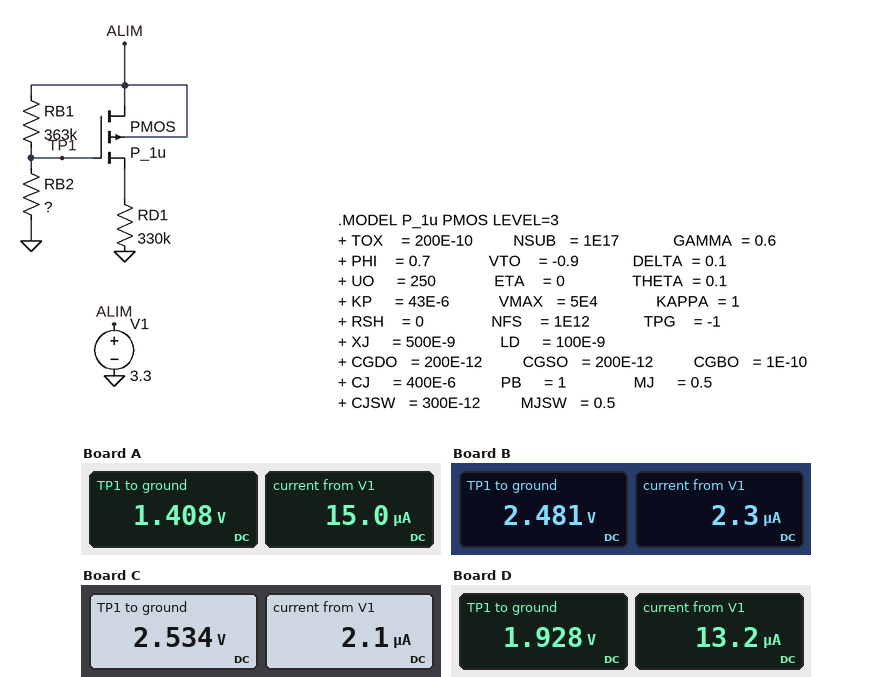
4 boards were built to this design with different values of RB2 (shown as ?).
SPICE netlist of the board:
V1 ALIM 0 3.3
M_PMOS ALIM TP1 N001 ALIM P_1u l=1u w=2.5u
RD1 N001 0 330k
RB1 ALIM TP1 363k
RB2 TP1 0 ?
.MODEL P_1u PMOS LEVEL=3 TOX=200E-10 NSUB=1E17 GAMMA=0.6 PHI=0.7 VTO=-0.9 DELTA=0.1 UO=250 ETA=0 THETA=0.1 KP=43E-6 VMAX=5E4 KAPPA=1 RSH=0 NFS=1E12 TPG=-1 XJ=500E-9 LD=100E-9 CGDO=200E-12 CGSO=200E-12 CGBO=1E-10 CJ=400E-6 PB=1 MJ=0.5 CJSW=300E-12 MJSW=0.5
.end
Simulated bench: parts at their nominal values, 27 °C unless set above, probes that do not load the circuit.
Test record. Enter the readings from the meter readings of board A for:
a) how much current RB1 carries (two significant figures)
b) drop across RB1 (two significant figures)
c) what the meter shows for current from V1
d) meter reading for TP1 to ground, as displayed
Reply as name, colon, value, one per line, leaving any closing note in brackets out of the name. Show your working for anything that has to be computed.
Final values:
how much current RB1 carries: (3.3 V - 1.408 V) / 363 kΩ = 5.2 µA
drop across RB1: 3.3 V - 1.408 V = 1.9 V
what the meter shows for current from V1: 15.0 µA
meter reading for TP1 to ground, as displayed: 1.408 V
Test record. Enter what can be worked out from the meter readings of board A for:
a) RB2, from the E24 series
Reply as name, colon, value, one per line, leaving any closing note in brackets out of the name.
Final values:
RB2, from the E24 series: 270 kΩ
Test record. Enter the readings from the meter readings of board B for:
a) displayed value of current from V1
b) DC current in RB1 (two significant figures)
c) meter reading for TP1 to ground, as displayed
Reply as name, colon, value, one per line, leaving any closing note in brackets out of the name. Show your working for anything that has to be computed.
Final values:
displayed value of current from V1: 2.3 µA
DC current in RB1: (3.3 V - 2.481 V) / 363 kΩ = 2.3 µA
meter reading for TP1 to ground, as displayed: 2.481 V
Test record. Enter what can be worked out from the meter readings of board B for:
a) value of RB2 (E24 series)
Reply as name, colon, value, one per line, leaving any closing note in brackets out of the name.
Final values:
value of RB2: 1.1 MΩ
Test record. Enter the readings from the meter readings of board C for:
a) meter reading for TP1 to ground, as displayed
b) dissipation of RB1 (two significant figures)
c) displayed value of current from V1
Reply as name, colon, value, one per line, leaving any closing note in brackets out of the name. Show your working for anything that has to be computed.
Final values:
meter reading for TP1 to ground, as displayed: 2.534 V
dissipation of RB1: (3.3 V - 2.534 V)^2 / 363 kΩ = 1.6 µW
displayed value of current from V1: 2.1 µA
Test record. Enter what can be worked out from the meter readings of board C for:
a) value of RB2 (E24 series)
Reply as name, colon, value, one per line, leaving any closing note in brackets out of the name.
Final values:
value of RB2: 1.2 MΩ
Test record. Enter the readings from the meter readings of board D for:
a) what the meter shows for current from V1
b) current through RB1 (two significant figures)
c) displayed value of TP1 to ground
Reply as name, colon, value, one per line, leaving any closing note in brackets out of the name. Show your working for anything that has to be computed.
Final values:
what the meter shows for current from V1: 13.2 µA
current through RB1: (3.3 V - 1.928 V) / 363 kΩ = 3.8 µA
displayed value of TP1 to ground: 1.928 V
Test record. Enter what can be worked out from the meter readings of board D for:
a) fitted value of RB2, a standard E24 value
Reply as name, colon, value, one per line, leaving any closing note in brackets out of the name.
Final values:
fitted value of RB2, a standard E24 value: 510 kΩ
